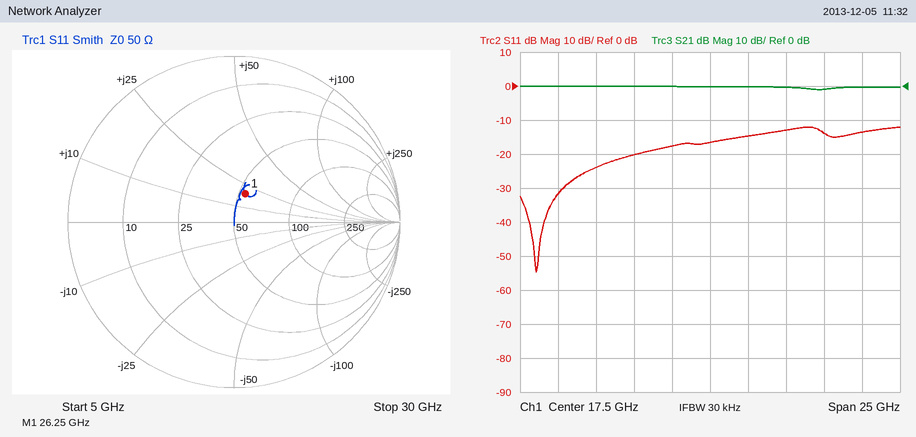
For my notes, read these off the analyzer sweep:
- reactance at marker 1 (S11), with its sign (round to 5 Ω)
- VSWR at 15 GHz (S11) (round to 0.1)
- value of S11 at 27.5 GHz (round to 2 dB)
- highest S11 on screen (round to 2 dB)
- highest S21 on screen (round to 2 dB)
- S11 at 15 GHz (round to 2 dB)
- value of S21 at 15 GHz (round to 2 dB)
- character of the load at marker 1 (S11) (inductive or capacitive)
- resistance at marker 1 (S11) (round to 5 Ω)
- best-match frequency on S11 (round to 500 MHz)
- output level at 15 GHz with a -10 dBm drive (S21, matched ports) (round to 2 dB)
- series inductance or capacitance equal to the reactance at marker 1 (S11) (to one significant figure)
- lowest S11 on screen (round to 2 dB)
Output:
+20 Ω
1.3
-14 dB
-12 dB
0 dB
-18 dB
0 dB
inductive
55 Ω
6.0 GHz
-10 dBm
100 pH
-54 dB
